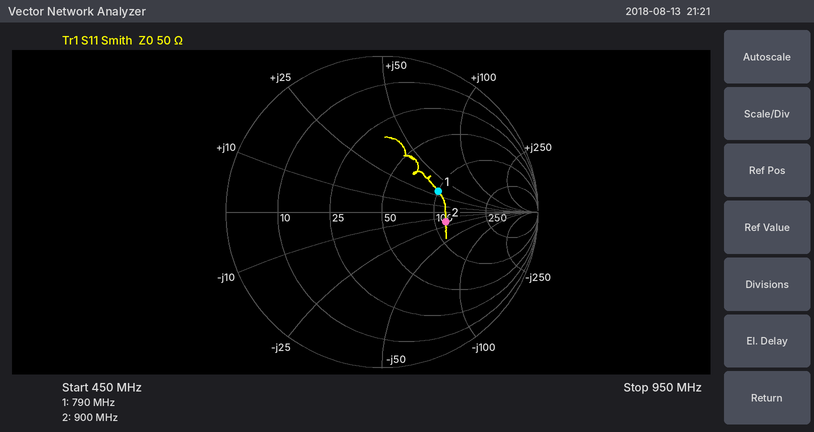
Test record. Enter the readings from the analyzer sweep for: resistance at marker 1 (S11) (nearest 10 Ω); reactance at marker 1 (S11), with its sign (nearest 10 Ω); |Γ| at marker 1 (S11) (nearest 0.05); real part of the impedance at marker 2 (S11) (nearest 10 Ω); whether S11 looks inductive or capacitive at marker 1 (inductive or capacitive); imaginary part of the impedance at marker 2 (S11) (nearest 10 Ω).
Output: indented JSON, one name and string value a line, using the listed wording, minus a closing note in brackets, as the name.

{
  "resistance at marker 1 (S11)": "100 Ω",
  "reactance at marker 1 (S11), with its sign": "+30 Ω",
  "|Γ| at marker 1 (S11)": "0.40",
  "real part of the impedance at marker 2 (S11)": "120 Ω",
  "whether S11 looks inductive or capacitive at marker 1": "inductive",
  "imaginary part of the impedance at marker 2 (S11)": "-20 Ω"
}
